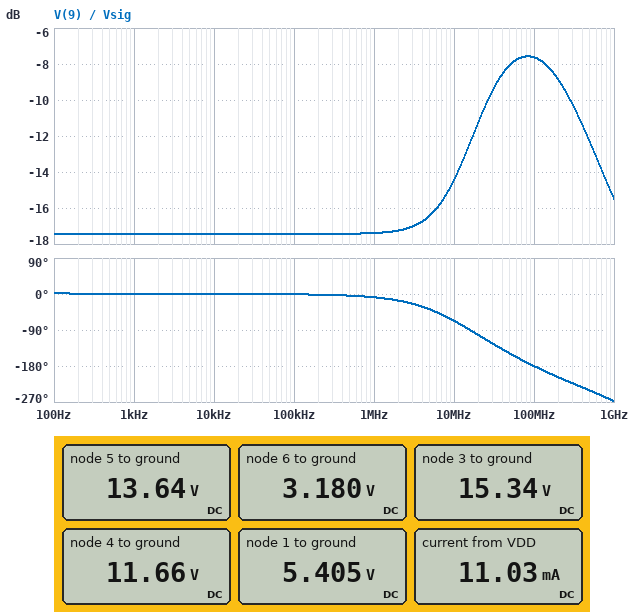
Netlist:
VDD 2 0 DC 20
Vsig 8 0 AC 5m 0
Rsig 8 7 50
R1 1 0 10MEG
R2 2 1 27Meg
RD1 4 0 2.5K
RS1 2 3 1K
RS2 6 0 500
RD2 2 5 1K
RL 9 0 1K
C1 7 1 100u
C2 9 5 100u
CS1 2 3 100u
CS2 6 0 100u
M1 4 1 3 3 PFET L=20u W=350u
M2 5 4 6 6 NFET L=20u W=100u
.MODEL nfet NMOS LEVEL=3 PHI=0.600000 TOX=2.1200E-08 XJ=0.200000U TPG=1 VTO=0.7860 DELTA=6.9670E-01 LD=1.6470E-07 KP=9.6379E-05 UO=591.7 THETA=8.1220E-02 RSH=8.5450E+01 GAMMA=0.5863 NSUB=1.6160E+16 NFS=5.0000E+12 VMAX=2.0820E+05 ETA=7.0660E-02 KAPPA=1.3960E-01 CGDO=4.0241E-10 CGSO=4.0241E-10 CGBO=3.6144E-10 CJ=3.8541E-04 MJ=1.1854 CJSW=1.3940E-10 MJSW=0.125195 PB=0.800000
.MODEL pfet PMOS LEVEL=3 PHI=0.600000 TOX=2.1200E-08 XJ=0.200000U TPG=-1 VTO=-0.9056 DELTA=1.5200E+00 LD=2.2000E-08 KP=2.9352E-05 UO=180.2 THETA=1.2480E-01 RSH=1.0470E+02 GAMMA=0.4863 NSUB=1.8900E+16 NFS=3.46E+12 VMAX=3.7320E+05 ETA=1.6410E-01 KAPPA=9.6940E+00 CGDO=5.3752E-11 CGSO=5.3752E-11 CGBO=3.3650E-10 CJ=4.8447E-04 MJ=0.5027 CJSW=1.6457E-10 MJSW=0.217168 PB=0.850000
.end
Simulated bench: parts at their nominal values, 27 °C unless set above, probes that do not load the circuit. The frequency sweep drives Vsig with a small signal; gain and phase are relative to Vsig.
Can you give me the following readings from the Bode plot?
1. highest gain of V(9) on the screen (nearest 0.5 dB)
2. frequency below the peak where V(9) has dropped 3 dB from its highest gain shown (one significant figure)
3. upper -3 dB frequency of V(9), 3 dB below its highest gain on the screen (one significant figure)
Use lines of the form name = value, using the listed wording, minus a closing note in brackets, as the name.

highest gain of V(9) on the screen = -7.5 dB
frequency below the peak where V(9) has dropped 3 dB from its highest gain shown = 20 MHz
upper -3 dB frequency of V(9), 3 dB below its highest gain on the screen = 300 MHz
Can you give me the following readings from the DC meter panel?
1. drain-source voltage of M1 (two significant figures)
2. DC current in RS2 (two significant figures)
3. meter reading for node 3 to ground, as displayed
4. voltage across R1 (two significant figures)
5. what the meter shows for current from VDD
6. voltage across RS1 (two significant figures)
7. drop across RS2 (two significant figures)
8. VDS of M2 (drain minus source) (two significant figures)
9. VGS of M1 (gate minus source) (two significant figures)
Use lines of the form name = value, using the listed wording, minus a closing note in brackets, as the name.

drain-source voltage of M1 = -3.7 V
DC current in RS2 = 6.4 mA
meter reading for node 3 to ground, as displayed = 15.34 V
voltage across R1 = 5.4 V
what the meter shows for current from VDD = 11.03 mA
voltage across RS1 = 4.7 V
drop across RS2 = 3.2 V
VDS of M2 (drain minus source) = 10 V
VGS of M1 (gate minus source) = -9.9 V
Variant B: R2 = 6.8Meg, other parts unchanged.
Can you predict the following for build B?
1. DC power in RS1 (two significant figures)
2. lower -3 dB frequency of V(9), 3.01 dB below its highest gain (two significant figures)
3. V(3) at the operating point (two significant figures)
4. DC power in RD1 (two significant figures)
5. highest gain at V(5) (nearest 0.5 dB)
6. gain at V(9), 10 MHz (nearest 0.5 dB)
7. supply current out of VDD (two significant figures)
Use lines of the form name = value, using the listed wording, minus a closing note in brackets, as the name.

DC power in RS1 = 6.9 mW
lower -3 dB frequency of V(9), 3.01 dB below its highest gain = 4.2 Hz
V(3) at the operating point = 17 V
DC power in RD1 = 17 mW
highest gain at V(5) = 1.0 dB
gain at V(9), 10 MHz = 0.5 dB
supply current out of VDD = 5.3 mA
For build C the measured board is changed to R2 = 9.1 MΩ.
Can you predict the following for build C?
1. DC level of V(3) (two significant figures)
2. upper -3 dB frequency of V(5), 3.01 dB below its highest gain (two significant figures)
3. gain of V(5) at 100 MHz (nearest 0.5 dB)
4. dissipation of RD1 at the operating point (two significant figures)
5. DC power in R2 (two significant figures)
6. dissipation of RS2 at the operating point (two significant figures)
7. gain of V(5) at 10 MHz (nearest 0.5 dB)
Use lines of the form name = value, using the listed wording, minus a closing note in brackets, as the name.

DC level of V(3) = 17 V
upper -3 dB frequency of V(5), 3.01 dB below its highest gain = 29 MHz
gain of V(5) at 100 MHz = -9.5 dB
dissipation of RD1 at the operating point = 28 mW
DC power in R2 = 10 µW
dissipation of RS2 at the operating point = 7.4 mW
gain of V(5) at 10 MHz = 2.5 dB
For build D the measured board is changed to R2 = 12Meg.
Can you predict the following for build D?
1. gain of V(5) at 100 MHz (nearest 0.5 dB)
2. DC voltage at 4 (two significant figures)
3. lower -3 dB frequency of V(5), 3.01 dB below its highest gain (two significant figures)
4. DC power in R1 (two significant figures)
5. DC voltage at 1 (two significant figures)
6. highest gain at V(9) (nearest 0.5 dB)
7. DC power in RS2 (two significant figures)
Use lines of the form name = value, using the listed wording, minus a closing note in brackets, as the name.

gain of V(5) at 100 MHz = -8.5 dB
DC voltage at 4 = 10 V
lower -3 dB frequency of V(5), 3.01 dB below its highest gain = 4.2 Hz
DC power in R1 = 8.3 µW
DC voltage at 1 = 9.1 V
highest gain at V(9) = 4.0 dB
DC power in RS2 = 13 mW
